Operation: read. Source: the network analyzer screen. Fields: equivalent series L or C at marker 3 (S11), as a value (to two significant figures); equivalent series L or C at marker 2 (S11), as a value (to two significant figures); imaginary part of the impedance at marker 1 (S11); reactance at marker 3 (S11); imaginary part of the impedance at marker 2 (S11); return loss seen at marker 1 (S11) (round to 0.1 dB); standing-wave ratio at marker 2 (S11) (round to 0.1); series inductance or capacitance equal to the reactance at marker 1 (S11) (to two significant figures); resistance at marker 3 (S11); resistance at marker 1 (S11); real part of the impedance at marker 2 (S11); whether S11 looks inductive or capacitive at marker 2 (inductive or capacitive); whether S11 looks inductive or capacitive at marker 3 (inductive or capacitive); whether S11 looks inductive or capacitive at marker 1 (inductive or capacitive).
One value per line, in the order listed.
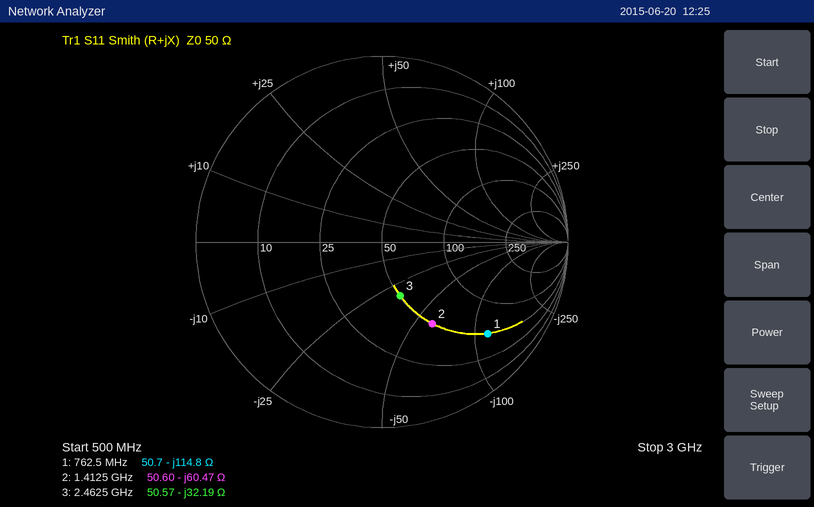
2.0 pF
1.9 pF
-114.8 Ω
-32.19 Ω
-60.47 Ω
2.5 dB
3.1
1.8 pF
50.57 Ω
50.7 Ω
50.60 Ω
capacitive
capacitive
capacitive
